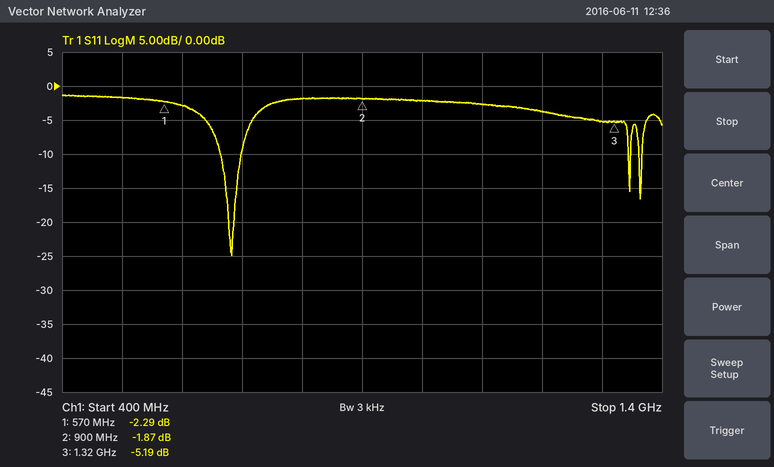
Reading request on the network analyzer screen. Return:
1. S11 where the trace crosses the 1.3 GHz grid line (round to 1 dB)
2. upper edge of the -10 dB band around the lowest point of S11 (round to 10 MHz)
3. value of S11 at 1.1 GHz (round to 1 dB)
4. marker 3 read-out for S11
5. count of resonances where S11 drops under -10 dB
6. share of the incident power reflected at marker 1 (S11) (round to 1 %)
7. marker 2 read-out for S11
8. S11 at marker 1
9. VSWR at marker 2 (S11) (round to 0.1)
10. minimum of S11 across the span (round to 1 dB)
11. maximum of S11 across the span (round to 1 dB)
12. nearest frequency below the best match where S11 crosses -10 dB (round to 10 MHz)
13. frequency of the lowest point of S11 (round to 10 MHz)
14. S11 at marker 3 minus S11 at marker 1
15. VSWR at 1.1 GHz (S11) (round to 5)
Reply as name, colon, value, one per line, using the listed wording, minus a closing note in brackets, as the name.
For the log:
S11 where the trace crosses the 1.3 GHz grid line: -5 dB
upper edge of the -10 dB band around the lowest point of S11: 700 MHz
value of S11 at 1.1 GHz: -3 dB
marker 3 read-out for S11: -5.19 dB
count of resonances where S11 drops under -10 dB: 3
share of the incident power reflected at marker 1 (S11): 59 %
marker 2 read-out for S11: -1.87 dB
S11 at marker 1: -2.29 dB
VSWR at marker 2 (S11): 9.3
minimum of S11 across the span: -25 dB
maximum of S11 across the span: -1 dB
nearest frequency below the best match where S11 crosses -10 dB: 660 MHz
frequency of the lowest point of S11: 680 MHz
S11 at marker 3 minus S11 at marker 1: -2.90 dB
VSWR at 1.1 GHz (S11): 5
